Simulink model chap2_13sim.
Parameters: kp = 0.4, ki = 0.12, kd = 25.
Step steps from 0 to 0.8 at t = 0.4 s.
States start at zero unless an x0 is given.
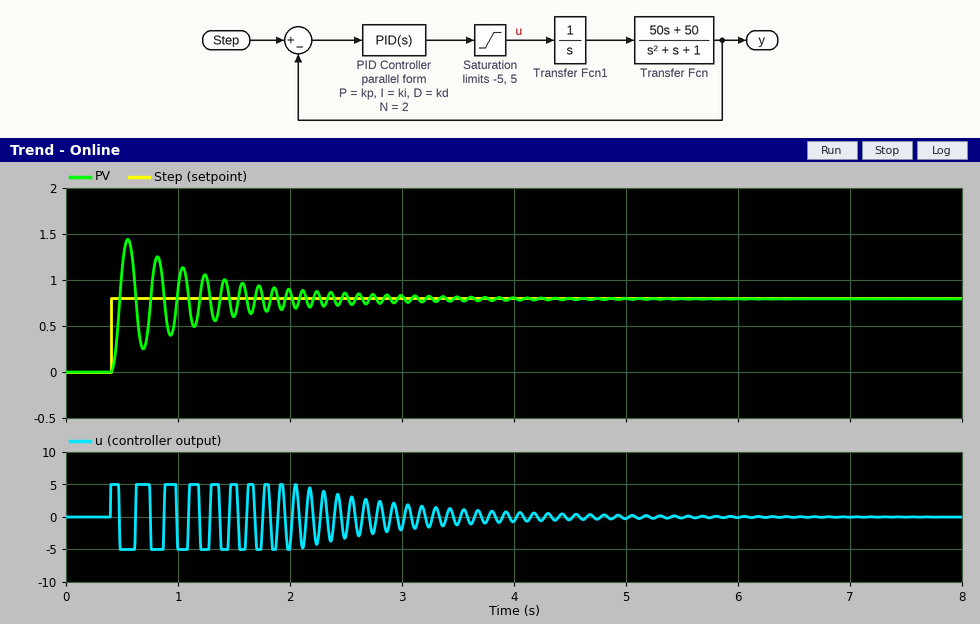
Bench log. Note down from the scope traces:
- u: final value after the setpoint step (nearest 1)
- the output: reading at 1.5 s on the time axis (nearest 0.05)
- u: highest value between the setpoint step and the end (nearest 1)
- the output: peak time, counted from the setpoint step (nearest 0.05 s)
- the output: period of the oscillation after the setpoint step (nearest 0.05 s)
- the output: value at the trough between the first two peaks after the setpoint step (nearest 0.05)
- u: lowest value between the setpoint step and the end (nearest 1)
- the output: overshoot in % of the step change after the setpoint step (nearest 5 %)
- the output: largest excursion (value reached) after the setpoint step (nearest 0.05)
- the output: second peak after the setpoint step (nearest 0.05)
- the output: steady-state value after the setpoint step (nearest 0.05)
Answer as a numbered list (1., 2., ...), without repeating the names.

1. 0
2. 0.60
3. 5
4. 0.15 s
5. 0.25 s
6. 0.25
7. -5
8. 80 %
9. 1.45
10. 1.25
11. 0.80
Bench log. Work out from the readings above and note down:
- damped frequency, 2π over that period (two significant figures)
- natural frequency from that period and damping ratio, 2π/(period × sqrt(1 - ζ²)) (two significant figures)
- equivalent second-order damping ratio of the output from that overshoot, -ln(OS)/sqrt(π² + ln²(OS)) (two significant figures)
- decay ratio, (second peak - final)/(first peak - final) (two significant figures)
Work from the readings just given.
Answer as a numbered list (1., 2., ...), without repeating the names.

1. 25 rad/s
2. 25 rad/s
3. 0.071
4. 0.69
